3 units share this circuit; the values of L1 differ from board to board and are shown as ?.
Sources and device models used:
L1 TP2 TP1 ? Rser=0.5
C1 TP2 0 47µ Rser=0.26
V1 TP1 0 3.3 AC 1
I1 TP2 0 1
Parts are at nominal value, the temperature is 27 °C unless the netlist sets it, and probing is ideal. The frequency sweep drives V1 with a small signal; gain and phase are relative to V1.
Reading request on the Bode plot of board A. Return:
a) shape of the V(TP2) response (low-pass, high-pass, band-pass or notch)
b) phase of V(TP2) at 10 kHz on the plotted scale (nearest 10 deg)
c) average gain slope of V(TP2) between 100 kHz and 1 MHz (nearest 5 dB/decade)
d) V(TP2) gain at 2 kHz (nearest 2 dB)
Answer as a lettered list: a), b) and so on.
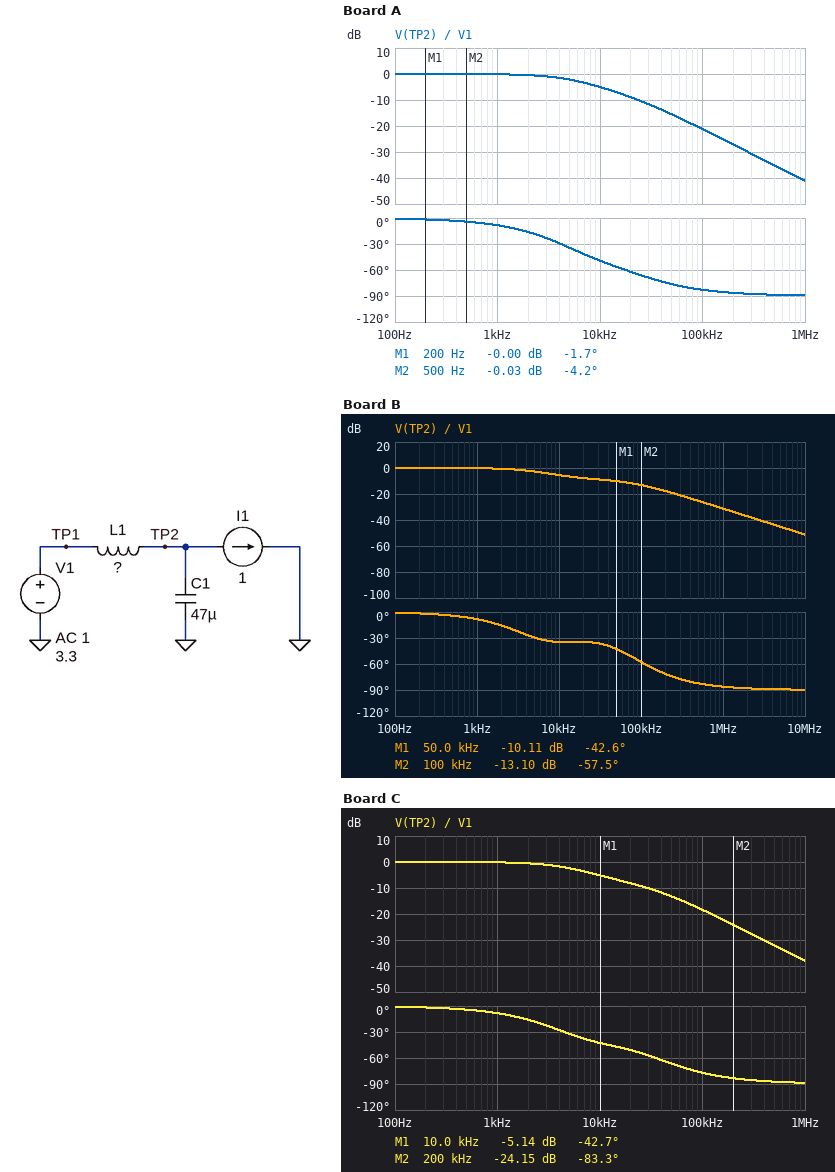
a) low-pass
b) -50 deg
c) -20 dB/decade
d) 0 dB
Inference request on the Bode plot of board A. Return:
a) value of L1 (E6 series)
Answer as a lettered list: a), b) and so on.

a) 4.7 µH
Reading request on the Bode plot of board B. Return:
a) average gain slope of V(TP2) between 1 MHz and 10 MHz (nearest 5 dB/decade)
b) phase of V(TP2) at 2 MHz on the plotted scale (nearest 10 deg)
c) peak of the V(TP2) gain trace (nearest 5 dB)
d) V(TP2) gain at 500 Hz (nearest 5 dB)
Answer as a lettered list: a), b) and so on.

a) -20 dB/decade
b) -90 deg
c) 0 dB
d) 0 dB
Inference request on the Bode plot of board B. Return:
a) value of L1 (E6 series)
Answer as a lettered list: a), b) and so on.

a) 1.5 µH
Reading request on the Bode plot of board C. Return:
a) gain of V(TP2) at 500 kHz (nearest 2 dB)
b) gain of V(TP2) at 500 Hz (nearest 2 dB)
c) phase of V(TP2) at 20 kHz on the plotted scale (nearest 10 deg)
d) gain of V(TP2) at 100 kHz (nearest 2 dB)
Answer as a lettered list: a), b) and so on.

a) -32 dB
b) 0 dB
c) -50 deg
d) -18 dB
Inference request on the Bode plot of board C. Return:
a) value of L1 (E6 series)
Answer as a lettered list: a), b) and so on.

a) 3.3 µH
